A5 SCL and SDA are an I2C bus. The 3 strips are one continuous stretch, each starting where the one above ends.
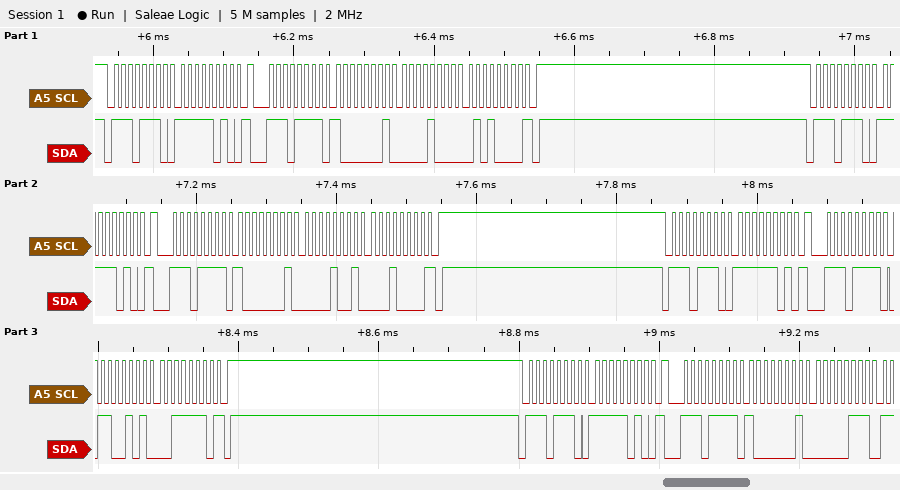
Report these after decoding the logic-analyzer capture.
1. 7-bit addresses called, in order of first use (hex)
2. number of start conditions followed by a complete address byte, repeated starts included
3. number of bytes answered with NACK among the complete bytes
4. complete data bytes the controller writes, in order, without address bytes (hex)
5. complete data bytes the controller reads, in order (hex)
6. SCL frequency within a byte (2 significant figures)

0x77
8
3
FA FA FD FA
81 08 50 81 09 10 65 3E 81 07
100 kHz
